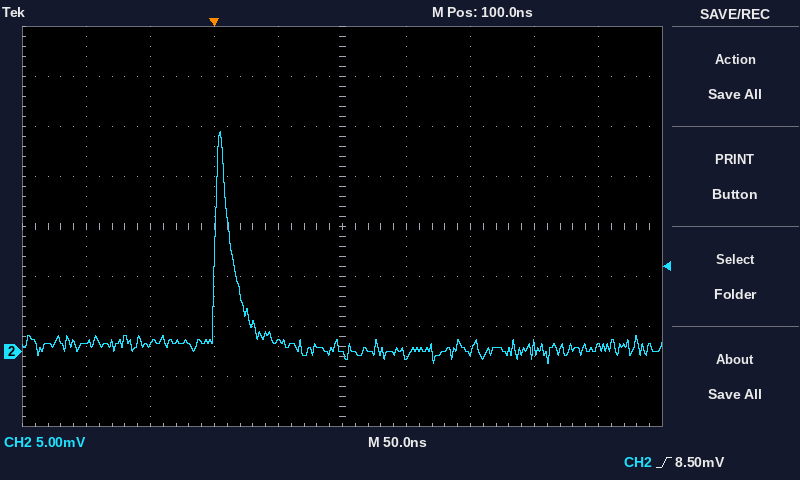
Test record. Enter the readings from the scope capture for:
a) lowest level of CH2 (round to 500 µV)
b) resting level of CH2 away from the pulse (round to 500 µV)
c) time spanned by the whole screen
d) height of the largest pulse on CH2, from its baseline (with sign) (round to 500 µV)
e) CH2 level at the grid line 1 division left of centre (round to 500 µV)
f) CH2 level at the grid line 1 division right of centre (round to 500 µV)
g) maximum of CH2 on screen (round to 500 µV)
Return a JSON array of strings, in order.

["-1.0 mV", "500 µV", "500 ns", "+21.5 mV", "1.0 mV", "-500 µV", "22.0 mV"]
